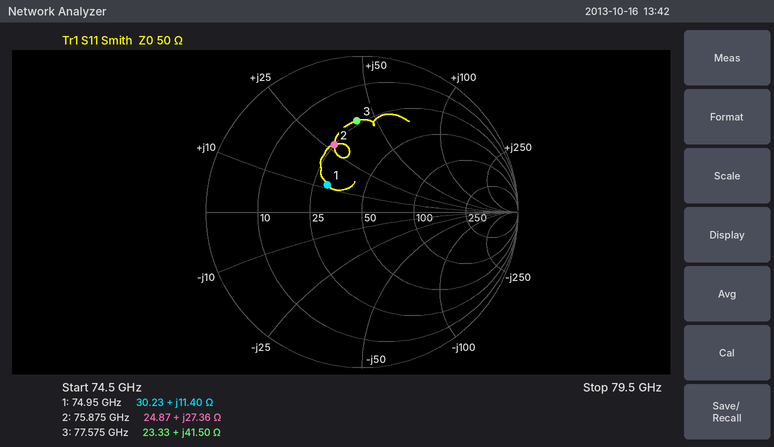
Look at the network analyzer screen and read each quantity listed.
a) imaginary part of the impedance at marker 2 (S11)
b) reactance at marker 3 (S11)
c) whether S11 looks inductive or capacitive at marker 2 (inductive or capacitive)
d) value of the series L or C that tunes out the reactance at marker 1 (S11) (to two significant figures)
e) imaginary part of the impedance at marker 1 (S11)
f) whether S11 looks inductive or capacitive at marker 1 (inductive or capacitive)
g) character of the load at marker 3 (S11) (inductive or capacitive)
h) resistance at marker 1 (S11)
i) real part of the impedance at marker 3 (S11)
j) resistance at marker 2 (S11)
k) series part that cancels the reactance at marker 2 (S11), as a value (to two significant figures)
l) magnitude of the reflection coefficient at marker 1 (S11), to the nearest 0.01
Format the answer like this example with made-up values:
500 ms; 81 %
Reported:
+27.36 Ω; +41.50 Ω; inductive; 190 fF; +11.40 Ω; inductive; inductive; 30.23 Ω; 23.33 Ω; 24.87 Ω; 77 fF; 0.28
